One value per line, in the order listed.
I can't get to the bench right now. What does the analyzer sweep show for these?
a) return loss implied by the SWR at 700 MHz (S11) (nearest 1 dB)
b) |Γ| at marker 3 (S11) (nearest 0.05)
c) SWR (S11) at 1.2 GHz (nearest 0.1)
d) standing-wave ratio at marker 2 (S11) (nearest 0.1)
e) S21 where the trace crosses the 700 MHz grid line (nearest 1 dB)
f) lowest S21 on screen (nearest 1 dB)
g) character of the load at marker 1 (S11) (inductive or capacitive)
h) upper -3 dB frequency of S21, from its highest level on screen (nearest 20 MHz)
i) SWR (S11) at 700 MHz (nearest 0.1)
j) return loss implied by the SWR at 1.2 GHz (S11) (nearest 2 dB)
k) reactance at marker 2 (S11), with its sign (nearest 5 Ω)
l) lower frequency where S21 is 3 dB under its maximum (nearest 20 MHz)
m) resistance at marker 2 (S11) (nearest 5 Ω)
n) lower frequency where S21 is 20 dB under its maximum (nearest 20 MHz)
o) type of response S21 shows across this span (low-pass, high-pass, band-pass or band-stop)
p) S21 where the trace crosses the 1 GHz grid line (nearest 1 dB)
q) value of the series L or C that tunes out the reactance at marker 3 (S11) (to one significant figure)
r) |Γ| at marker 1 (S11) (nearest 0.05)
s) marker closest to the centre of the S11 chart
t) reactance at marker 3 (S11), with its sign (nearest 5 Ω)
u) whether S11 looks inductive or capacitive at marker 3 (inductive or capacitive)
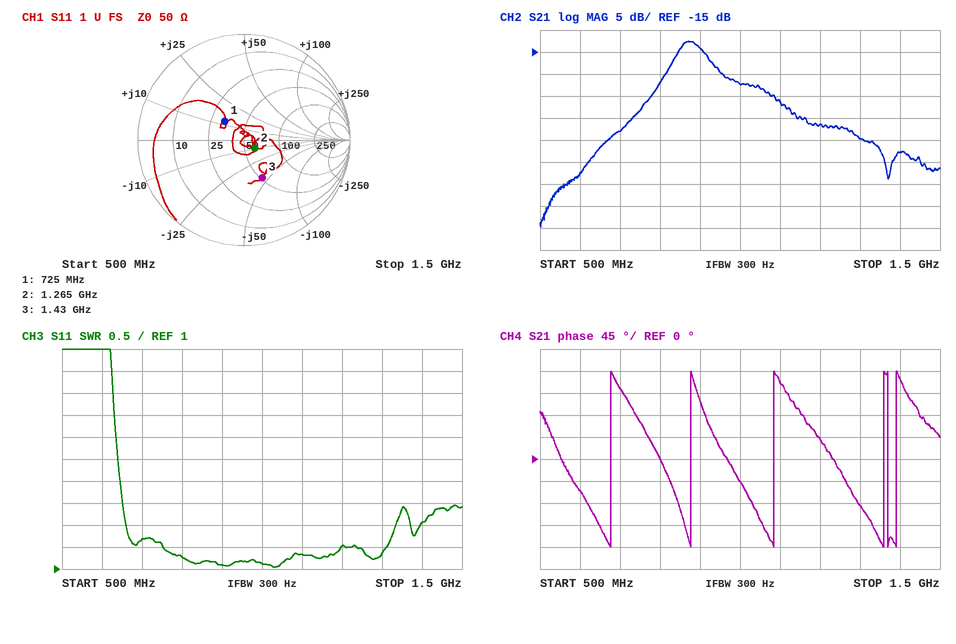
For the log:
12 dB
0.40
1.5
1.3
-33 dB
-55 dB
inductive
920 MHz
1.7
14 dB
-10 Ω
840 MHz
60 Ω
700 MHz
band-pass
-22 dB
5 nH
0.25
marker 2
-45 Ω
capacitive
